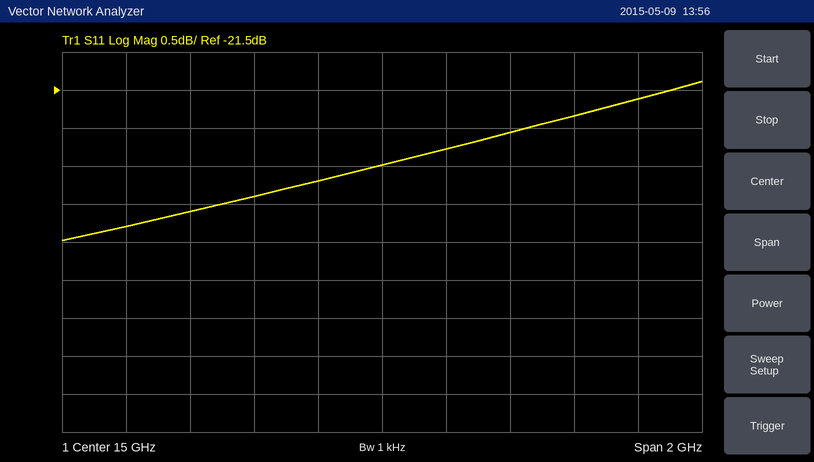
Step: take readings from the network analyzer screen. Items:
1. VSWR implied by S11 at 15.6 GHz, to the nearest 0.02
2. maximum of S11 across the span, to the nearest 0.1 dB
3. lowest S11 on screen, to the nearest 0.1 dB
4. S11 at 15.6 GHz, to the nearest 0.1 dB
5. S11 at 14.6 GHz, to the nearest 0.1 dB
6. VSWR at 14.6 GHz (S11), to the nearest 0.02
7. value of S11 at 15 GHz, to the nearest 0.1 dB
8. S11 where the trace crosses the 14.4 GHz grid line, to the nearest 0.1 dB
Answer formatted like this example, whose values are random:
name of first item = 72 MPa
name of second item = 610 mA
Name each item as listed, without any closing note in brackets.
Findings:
VSWR implied by S11 at 15.6 GHz, to the nearest 0.02 = 1.18
maximum of S11 across the span, to the nearest 0.1 dB = -21.4 dB
lowest S11 on screen, to the nearest 0.1 dB = -23.5 dB
S11 at 15.6 GHz, to the nearest 0.1 dB = -21.8 dB
S11 at 14.6 GHz, to the nearest 0.1 dB = -22.9 dB
VSWR at 14.6 GHz (S11), to the nearest 0.02 = 1.16
value of S11 at 15 GHz, to the nearest 0.1 dB = -22.5 dB
S11 where the trace crosses the 14.4 GHz grid line, to the nearest 0.1 dB = -23.1 dB
